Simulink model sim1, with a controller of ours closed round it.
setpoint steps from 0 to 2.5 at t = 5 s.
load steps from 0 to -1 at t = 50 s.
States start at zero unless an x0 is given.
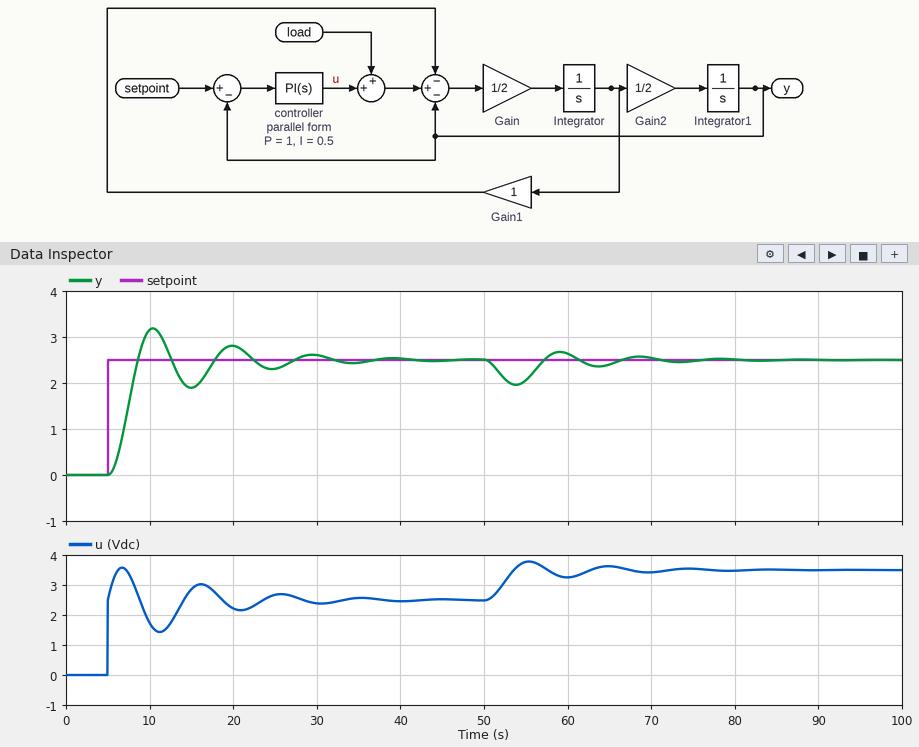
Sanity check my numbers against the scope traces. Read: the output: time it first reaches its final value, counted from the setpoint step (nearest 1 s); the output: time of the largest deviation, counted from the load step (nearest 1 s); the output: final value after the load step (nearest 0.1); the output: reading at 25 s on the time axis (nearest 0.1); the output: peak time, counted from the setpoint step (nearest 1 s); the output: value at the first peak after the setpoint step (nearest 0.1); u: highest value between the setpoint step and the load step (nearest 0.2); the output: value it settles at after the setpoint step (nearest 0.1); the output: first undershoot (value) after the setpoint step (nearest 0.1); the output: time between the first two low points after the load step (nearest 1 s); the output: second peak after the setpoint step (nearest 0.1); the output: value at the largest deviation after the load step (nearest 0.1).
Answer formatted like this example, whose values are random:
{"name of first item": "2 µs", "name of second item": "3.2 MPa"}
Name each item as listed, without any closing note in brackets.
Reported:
{"the output: time it first reaches its final value, counted from the setpoint step": "4 s", "the output: time of the largest deviation, counted from the load step": "4 s", "the output: final value after the load step": "2.5", "the output: reading at 25 s on the time axis": "2.3", "the output: peak time, counted from the setpoint step": "5 s", "the output: value at the first peak after the setpoint step": "3.2", "u: highest value between the setpoint step and the load step": "3.6", "the output: value it settles at after the setpoint step": "2.5", "the output: first undershoot (value) after the setpoint step": "1.9", "the output: time between the first two low points after the load step": "10 s", "the output: second peak after the setpoint step": "2.8", "the output: value at the largest deviation after the load step": "2.0"}
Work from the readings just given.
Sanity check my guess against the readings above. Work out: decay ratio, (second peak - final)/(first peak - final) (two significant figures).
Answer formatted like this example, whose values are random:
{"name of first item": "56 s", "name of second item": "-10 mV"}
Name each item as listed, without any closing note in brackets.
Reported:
{"decay ratio, (second peak - final)/(first peak - final)": "0.43"}
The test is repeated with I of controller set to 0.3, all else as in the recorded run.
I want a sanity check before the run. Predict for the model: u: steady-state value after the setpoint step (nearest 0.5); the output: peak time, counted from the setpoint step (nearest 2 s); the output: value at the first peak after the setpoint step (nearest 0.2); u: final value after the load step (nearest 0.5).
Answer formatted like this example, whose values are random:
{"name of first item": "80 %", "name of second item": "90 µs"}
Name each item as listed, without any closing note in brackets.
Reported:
{"u: steady-state value after the setpoint step": "2.5", "the output: peak time, counted from the setpoint step": "6 s", "the output: value at the first peak after the setpoint step": "2.6", "u: final value after the load step": "3.5"}
